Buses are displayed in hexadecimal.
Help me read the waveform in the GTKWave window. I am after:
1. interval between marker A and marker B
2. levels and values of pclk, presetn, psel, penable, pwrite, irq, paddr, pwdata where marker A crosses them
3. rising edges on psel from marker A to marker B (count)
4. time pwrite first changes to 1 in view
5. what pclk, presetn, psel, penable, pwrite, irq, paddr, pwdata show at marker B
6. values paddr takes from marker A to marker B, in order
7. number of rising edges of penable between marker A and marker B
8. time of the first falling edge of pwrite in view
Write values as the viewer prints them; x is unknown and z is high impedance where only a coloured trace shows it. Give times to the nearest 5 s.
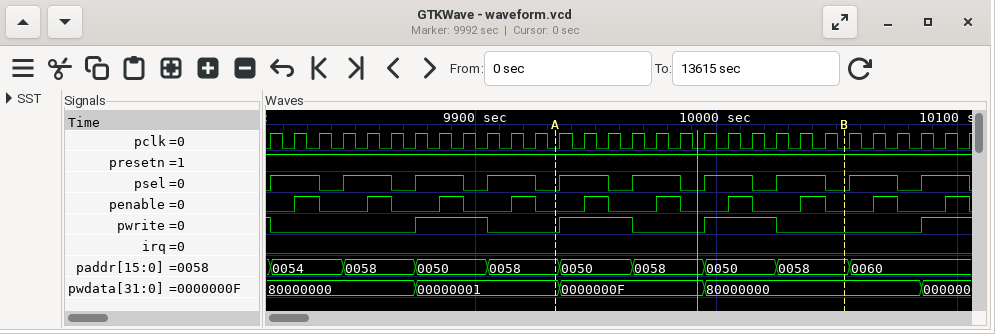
120 s
pclk=0, presetn=1, psel=0, penable=0, pwrite=0, irq=0, paddr=0058, pwdata=00000001
4
9875 s
pclk=0, presetn=1, psel=0, penable=0, pwrite=0, irq=0, paddr=0058, pwdata=80000000
0058, 0050, 0058, 0050, 0058
4
9815 s
